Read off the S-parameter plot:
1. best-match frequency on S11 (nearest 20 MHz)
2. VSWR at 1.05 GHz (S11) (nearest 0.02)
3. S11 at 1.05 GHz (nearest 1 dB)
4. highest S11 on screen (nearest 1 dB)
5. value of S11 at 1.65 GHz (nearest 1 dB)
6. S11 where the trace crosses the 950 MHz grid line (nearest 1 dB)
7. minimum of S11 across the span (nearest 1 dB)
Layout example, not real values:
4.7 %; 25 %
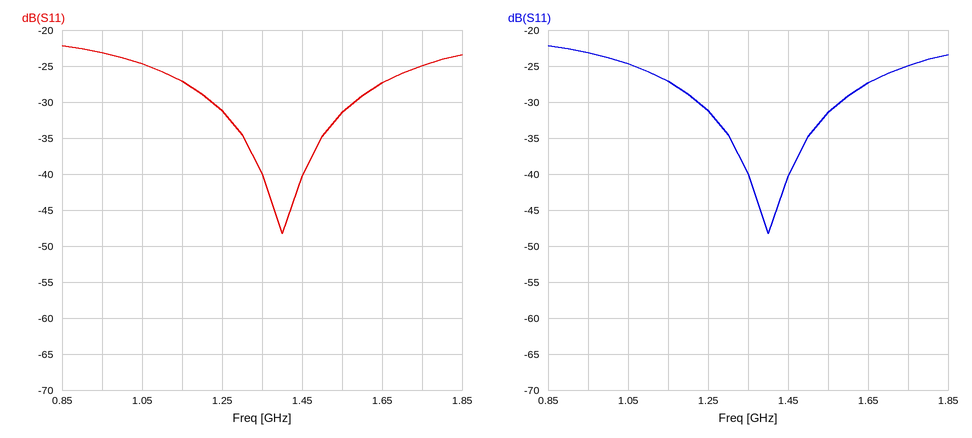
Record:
1.40 GHz; 1.12; -25 dB; -22 dB; -27 dB; -23 dB; -48 dB
